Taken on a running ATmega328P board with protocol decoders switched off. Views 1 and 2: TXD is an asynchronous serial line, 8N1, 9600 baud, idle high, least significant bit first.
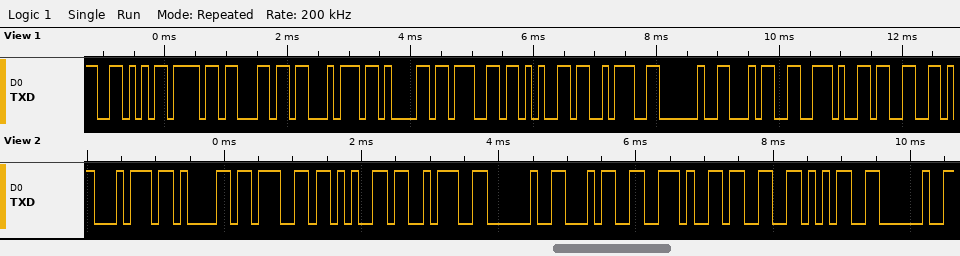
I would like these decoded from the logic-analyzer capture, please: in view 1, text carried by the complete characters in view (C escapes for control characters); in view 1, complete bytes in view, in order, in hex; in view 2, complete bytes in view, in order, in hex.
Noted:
"Voltage: 4.3"
0x56 0x6F 0x6C 0x74 0x61 0x67 0x65 0x3A 0x20 0x34 0x2E 0x33
0x74 0x61 0x67 0x65 0x3A 0x20 0x34 0x2E 0x33 0x35 0x20
